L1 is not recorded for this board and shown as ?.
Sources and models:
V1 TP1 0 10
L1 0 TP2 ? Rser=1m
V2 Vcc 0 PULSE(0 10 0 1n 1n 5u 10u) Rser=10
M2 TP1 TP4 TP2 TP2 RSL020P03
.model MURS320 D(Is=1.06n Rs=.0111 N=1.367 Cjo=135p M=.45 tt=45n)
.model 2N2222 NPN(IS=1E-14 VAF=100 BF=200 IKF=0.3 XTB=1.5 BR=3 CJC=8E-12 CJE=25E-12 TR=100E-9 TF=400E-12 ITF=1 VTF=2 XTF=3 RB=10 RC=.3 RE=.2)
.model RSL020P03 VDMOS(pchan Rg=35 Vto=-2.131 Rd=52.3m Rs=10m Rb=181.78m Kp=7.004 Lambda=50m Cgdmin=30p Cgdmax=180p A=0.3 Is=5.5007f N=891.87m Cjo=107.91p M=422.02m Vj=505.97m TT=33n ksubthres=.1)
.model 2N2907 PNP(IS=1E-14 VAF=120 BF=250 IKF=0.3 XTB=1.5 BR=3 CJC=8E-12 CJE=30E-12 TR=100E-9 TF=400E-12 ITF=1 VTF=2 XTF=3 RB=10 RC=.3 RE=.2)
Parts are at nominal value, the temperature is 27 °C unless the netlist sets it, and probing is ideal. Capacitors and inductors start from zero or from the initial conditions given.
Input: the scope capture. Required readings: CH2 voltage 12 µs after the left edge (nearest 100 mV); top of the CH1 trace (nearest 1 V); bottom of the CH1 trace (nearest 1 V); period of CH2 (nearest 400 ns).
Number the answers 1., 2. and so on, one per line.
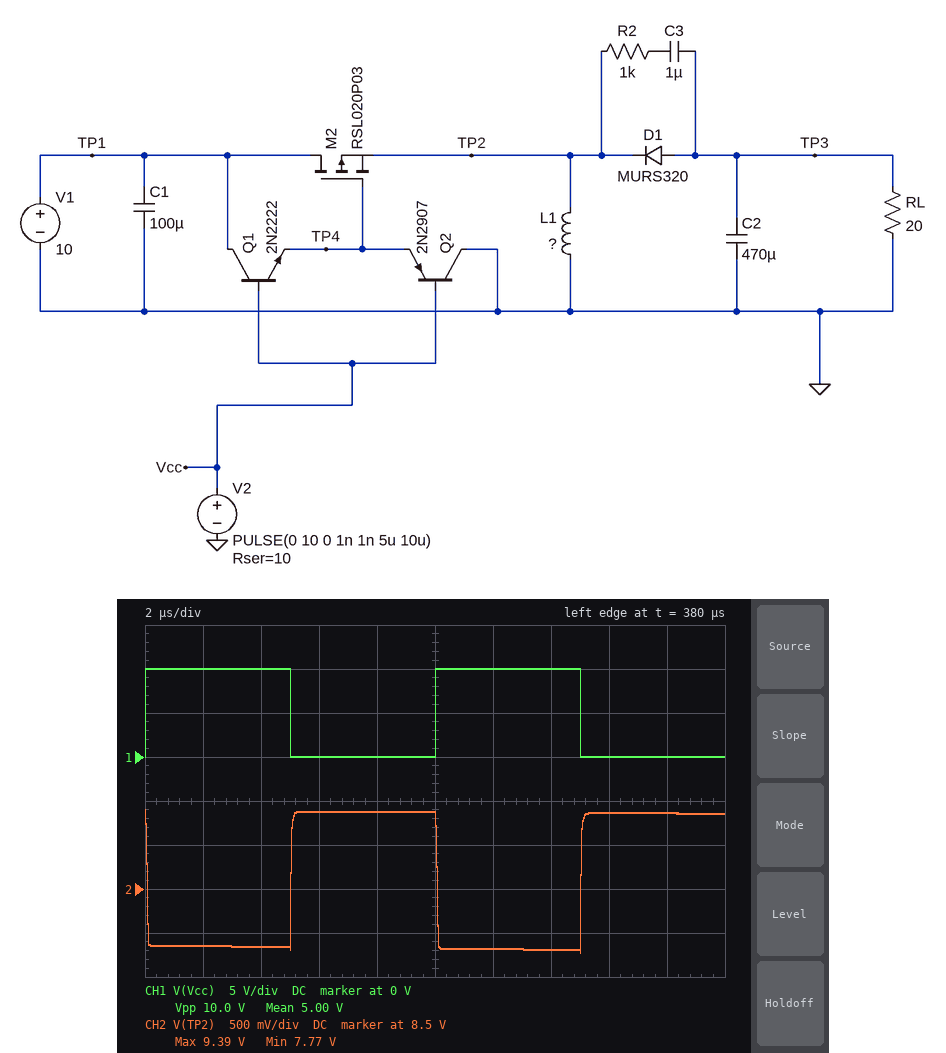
1. 7.8 V
2. 10 V
3. 0 V
4. 10.0 µs
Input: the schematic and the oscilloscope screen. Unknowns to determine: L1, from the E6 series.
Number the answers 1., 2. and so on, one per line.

1. 470 µH
